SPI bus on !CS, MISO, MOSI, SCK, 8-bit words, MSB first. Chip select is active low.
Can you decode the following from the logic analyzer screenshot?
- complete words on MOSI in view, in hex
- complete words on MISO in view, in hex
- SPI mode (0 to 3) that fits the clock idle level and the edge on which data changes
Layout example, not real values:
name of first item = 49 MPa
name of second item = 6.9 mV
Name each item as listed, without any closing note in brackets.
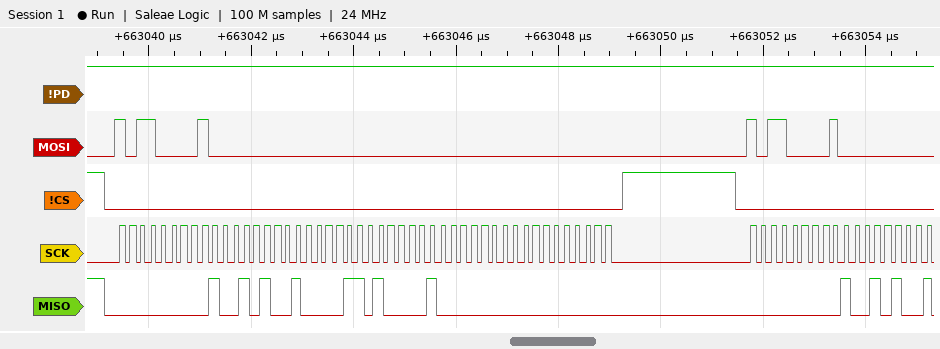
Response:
complete words on MOSI in view, in hex = B0, 80, 00, 00, 00, 00, B0, 80
complete words on MISO in view, in hex = 00, 4A, 43, 42, 00, 00, 00, 4A
SPI mode (0 to 3) that fits the clock idle level and the edge on which data changes = 0
